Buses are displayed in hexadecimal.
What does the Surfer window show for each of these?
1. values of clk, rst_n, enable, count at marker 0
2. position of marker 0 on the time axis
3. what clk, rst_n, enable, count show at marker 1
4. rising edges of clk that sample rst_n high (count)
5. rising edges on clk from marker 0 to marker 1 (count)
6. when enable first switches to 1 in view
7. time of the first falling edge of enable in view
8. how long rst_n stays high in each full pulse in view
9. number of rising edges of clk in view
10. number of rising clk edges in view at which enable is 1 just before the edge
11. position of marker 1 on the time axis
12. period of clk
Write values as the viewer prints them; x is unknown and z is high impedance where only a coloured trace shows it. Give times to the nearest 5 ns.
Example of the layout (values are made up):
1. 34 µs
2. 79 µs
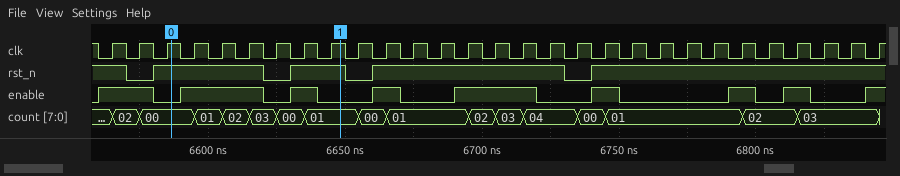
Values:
1. clk=1, rst_n=1, enable=0, count=00
2. 6585 ns
3. clk=1, rst_n=1, enable=0, count=01
4. 25
5. 6
6. 6560 ns
7. 6580 ns
8. 40 ns, 20 ns, 70 ns
9. 29
10. 14
11. 6650 ns
12. 10 ns
